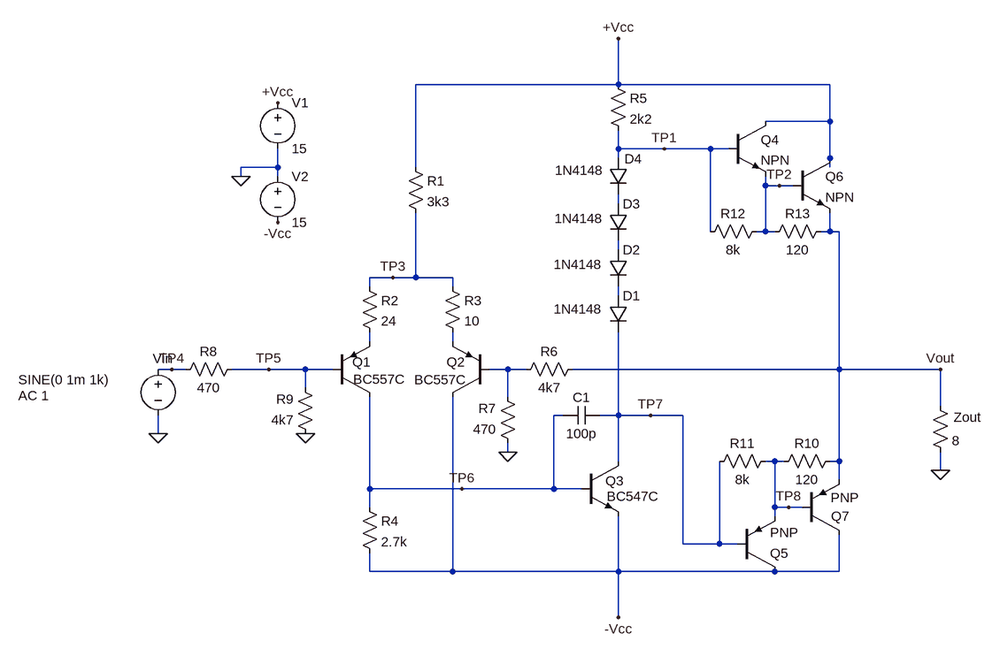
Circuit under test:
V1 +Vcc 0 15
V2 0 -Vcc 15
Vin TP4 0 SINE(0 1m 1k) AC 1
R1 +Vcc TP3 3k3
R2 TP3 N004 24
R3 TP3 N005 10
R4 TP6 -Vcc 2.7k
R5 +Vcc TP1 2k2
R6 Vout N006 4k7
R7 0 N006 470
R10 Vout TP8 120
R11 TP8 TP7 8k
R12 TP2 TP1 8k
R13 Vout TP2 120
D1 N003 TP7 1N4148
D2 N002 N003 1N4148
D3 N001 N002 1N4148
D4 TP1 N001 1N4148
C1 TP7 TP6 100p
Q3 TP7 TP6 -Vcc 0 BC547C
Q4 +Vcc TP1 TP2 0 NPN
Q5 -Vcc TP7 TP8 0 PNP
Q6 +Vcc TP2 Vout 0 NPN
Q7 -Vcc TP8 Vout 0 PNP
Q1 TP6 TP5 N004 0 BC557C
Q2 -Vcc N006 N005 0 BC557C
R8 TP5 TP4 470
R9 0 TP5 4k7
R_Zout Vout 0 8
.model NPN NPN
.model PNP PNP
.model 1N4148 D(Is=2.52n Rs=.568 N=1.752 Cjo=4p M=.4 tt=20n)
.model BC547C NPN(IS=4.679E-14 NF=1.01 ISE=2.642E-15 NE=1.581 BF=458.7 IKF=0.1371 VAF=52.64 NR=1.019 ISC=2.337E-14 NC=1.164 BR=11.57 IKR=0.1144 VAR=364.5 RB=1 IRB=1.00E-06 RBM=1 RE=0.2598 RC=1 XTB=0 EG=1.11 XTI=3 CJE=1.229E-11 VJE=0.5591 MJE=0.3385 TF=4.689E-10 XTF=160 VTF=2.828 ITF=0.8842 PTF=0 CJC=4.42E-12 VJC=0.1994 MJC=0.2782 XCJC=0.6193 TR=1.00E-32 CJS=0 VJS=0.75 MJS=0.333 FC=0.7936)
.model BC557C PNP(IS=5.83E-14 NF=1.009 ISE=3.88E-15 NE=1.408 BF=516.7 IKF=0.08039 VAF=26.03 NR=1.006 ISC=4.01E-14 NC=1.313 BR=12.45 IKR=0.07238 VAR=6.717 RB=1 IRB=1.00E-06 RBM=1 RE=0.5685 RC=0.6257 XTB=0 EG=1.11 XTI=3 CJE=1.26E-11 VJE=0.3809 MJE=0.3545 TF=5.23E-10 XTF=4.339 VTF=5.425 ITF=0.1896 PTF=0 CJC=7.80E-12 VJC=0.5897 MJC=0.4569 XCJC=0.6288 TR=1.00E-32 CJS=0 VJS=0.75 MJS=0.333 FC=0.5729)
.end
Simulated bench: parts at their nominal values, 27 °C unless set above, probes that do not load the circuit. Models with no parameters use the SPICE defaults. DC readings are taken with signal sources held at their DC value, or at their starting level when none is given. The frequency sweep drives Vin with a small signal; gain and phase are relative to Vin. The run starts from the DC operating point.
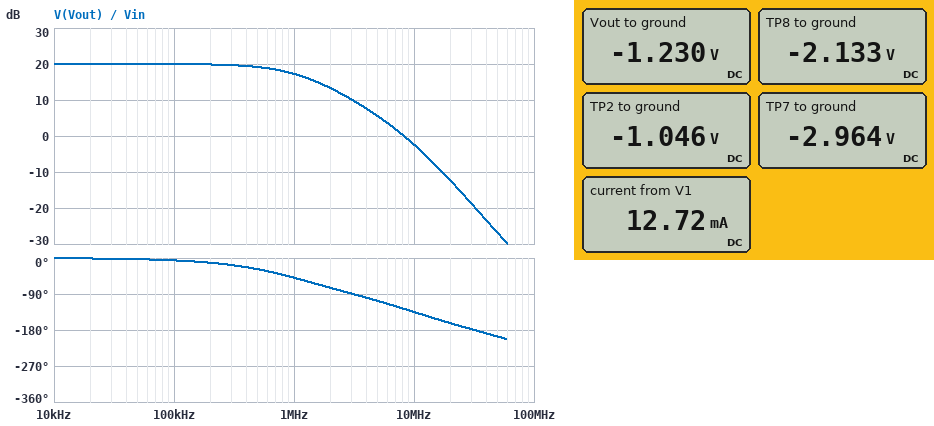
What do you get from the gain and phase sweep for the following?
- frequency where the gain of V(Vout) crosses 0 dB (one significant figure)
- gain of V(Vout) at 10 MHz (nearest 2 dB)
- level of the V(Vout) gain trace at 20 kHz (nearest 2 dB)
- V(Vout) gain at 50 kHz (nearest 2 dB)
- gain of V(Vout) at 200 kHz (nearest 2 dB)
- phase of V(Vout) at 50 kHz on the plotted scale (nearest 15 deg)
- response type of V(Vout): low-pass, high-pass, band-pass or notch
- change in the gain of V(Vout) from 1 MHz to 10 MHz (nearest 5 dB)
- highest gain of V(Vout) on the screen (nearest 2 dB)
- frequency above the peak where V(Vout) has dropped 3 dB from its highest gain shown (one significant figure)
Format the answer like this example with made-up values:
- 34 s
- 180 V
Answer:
- 8 MHz
- -2 dB
- 20 dB
- 20 dB
- 20 dB
- 0 deg
- low-pass
- -20 dB
- 20 dB
- 1 MHz
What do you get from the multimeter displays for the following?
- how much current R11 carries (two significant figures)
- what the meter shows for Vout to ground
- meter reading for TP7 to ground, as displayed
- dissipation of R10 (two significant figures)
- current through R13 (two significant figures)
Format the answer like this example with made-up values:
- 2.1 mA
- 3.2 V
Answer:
- 100 µA
- -1.230 V
- -2.964 V
- 6.8 mW
- 1.5 mA
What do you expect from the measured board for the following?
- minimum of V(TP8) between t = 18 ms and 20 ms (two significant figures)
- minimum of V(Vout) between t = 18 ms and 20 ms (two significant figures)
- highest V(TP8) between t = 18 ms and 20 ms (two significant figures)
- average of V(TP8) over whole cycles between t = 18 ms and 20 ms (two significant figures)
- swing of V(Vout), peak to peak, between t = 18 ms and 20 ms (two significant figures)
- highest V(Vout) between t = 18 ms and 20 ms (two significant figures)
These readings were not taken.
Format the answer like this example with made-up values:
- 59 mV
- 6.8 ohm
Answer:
- -2.1 V
- -1.2 V
- -2.1 V
- -2.1 V
- 20 mV
- -1.2 V
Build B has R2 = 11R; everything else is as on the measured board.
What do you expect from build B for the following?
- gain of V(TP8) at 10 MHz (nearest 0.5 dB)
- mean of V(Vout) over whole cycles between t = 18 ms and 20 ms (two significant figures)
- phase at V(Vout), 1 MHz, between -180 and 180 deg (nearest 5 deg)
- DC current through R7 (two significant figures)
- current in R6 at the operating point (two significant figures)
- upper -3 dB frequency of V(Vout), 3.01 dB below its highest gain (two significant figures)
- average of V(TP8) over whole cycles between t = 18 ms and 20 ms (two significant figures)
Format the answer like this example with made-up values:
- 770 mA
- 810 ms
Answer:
- -1.5 dB
- -1.3 V
- -45 deg
- 240 µA
- 250 µA
- 1.2 MHz
- -2.2 V
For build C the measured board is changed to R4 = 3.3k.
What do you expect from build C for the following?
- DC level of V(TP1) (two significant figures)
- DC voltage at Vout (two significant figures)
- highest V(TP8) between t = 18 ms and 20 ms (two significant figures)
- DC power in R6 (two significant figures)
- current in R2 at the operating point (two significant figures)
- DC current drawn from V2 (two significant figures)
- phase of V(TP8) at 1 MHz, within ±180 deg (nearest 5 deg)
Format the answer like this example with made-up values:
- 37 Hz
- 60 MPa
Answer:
- -340 mV
- -1.3 V
- -2.2 V
- 300 µW
- 220 µA
- 180 mA
- -55 deg
